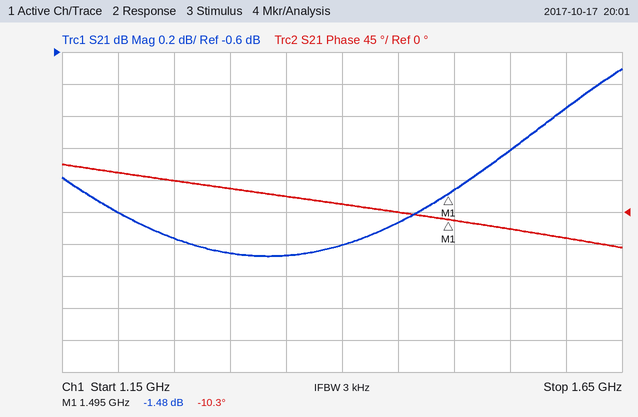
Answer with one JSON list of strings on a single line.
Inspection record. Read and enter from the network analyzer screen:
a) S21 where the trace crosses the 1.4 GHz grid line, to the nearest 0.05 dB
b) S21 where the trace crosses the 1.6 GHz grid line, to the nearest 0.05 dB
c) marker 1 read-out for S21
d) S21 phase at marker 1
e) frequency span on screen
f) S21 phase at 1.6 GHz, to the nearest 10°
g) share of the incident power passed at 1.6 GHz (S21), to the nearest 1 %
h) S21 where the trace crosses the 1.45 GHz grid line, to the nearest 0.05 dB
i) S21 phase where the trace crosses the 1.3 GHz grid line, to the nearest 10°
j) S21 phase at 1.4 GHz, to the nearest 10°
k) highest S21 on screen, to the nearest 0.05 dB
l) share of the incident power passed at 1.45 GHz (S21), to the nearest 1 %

["-1.80 dB", "-0.95 dB", "-1.48 dB", "-10.3°", "500 MHz", "-40°", "80 %", "-1.65 dB", "30°", "10°", "-0.70 dB", "68 %"]
